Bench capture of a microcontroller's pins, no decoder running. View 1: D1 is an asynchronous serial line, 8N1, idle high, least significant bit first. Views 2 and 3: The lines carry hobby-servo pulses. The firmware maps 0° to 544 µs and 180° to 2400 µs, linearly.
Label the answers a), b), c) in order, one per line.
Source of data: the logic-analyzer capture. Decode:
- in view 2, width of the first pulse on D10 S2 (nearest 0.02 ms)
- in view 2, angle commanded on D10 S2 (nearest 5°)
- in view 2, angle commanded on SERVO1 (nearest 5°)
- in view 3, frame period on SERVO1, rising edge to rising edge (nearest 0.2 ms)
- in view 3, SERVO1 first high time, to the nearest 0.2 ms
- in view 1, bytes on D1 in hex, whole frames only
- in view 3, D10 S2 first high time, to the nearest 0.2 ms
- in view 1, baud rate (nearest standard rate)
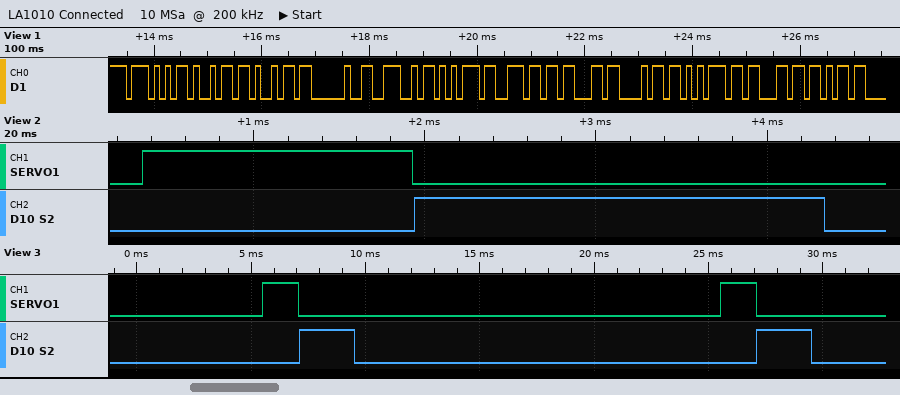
a) 2.40 ms
b) 180°
c) 100°
d) 20.0 ms
e) 1.6 ms
f) 0x57 0x69 0x69 0x20 0x4E 0x75 0x6E 0x63 0x68 0x75 0x63 0x6B
g) 2.4 ms
h) 9600 baud
